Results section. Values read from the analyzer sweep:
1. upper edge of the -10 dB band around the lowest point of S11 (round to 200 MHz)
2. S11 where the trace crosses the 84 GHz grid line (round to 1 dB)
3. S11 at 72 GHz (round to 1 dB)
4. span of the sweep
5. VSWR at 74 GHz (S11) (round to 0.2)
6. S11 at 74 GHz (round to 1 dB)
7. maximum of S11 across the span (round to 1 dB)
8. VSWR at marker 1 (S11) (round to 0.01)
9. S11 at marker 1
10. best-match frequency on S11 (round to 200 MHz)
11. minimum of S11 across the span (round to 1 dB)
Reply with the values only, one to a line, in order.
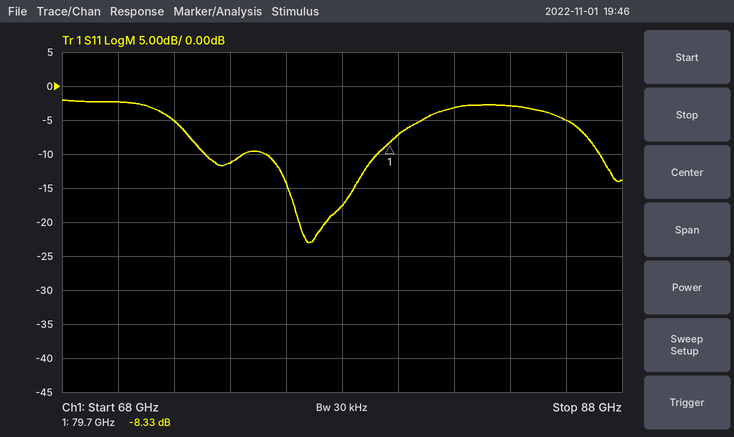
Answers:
79.2 GHz
-3 dB
-5 dB
20 GHz
1.8
-11 dB
-2 dB
2.24
-8.33 dB
76.8 GHz
-23 dB
